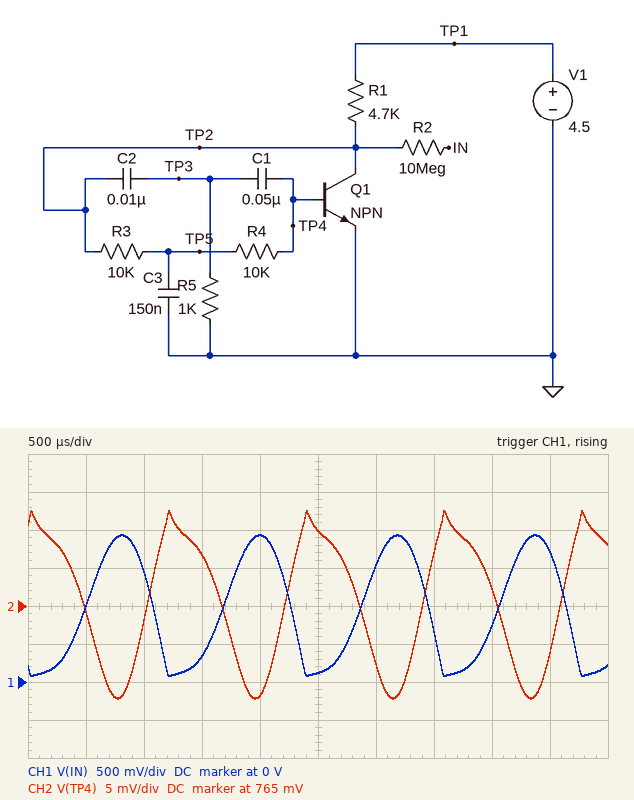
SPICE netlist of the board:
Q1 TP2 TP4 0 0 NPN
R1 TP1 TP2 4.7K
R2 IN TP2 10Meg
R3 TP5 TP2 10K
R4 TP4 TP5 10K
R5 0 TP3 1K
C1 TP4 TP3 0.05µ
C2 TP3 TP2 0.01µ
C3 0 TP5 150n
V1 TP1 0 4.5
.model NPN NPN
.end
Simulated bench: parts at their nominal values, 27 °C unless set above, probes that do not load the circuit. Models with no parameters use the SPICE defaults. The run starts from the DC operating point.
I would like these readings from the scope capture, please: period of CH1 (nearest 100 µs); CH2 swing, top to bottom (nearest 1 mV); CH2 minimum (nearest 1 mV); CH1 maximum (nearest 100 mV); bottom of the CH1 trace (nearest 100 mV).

1.2 ms
25 mV
753 mV
1.9 V
100 mV
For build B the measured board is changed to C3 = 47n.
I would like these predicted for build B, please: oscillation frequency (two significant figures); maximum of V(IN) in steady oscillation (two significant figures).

1.2 kHz
2.0 V
